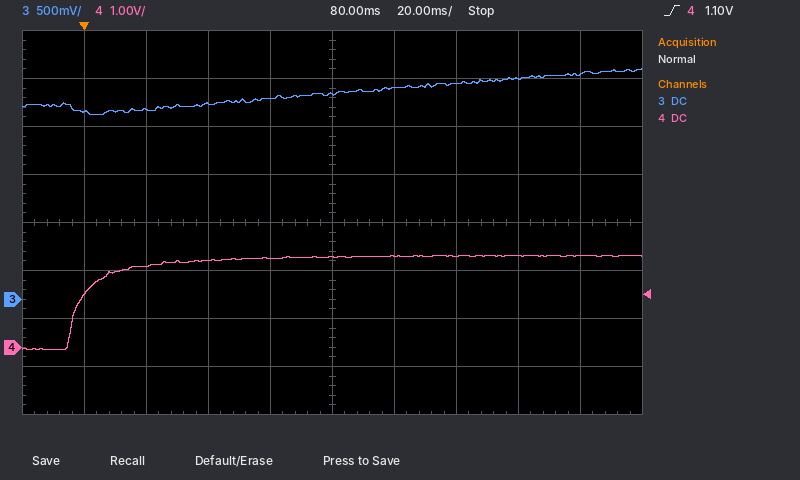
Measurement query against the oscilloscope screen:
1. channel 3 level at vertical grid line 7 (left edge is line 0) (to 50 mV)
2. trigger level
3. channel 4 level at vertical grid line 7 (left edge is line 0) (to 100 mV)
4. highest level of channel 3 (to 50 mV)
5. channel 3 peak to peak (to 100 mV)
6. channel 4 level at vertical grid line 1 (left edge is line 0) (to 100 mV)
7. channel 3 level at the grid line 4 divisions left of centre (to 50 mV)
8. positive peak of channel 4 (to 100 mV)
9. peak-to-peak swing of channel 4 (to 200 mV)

2.25 V
1.10 V
1.9 V
2.40 V
500 mV
1.1 V
1.95 V
1.9 V
2.0 V
